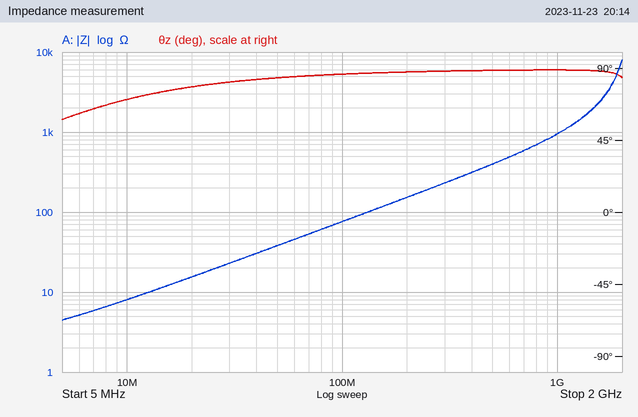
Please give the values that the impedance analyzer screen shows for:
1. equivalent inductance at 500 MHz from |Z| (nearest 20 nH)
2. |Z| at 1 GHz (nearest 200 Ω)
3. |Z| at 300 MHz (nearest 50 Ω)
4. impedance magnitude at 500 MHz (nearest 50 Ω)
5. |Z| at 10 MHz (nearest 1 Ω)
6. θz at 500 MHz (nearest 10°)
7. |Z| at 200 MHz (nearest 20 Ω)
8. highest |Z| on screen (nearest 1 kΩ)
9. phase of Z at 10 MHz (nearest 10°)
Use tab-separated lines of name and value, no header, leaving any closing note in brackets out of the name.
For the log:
equivalent inductance at 500 MHz from |Z|	120 nH
|Z| at 1 GHz	1.0 kΩ
|Z| at 300 MHz	250 Ω
impedance magnitude at 500 MHz	400 Ω
|Z| at 10 MHz	8 Ω
θz at 500 MHz	90°
|Z| at 200 MHz	160 Ω
highest |Z| on screen	8 kΩ
phase of Z at 10 MHz	70°
